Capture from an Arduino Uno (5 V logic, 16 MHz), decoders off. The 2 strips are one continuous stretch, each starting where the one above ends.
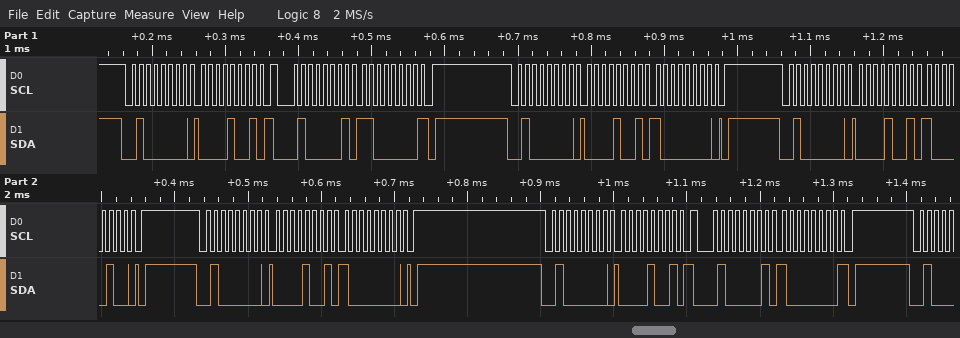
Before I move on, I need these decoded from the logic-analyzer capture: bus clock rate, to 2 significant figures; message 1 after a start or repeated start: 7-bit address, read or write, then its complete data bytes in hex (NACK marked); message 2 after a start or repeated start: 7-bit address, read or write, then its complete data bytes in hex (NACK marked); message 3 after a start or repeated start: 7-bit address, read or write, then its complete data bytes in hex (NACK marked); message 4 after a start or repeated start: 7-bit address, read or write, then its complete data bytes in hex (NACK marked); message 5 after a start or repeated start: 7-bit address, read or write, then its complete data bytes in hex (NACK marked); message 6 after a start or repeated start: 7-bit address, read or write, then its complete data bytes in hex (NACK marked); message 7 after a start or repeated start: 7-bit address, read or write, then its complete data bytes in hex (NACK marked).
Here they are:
100 kHz
0x20 write: 09
0x20 read: C0 NACK
0x20 write: 09 80
0x20 write: 09 84
0x20 write: 09 80
0x20 write: 09
0x20 read: 80 NACK
